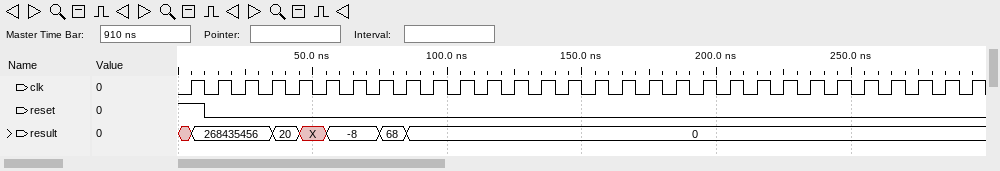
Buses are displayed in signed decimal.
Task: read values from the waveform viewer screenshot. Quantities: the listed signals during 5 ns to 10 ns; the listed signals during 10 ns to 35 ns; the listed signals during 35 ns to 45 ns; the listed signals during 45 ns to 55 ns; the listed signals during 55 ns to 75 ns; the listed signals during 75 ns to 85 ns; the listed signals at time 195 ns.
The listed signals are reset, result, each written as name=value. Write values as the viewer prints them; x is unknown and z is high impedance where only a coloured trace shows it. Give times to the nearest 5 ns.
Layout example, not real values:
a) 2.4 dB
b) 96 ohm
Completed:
a) reset=1, result=268435456
b) reset=0, result=268435456
c) reset=0, result=20
d) reset=0, result=X
e) reset=0, result=-8
f) reset=0, result=68
g) reset=0, result=0
